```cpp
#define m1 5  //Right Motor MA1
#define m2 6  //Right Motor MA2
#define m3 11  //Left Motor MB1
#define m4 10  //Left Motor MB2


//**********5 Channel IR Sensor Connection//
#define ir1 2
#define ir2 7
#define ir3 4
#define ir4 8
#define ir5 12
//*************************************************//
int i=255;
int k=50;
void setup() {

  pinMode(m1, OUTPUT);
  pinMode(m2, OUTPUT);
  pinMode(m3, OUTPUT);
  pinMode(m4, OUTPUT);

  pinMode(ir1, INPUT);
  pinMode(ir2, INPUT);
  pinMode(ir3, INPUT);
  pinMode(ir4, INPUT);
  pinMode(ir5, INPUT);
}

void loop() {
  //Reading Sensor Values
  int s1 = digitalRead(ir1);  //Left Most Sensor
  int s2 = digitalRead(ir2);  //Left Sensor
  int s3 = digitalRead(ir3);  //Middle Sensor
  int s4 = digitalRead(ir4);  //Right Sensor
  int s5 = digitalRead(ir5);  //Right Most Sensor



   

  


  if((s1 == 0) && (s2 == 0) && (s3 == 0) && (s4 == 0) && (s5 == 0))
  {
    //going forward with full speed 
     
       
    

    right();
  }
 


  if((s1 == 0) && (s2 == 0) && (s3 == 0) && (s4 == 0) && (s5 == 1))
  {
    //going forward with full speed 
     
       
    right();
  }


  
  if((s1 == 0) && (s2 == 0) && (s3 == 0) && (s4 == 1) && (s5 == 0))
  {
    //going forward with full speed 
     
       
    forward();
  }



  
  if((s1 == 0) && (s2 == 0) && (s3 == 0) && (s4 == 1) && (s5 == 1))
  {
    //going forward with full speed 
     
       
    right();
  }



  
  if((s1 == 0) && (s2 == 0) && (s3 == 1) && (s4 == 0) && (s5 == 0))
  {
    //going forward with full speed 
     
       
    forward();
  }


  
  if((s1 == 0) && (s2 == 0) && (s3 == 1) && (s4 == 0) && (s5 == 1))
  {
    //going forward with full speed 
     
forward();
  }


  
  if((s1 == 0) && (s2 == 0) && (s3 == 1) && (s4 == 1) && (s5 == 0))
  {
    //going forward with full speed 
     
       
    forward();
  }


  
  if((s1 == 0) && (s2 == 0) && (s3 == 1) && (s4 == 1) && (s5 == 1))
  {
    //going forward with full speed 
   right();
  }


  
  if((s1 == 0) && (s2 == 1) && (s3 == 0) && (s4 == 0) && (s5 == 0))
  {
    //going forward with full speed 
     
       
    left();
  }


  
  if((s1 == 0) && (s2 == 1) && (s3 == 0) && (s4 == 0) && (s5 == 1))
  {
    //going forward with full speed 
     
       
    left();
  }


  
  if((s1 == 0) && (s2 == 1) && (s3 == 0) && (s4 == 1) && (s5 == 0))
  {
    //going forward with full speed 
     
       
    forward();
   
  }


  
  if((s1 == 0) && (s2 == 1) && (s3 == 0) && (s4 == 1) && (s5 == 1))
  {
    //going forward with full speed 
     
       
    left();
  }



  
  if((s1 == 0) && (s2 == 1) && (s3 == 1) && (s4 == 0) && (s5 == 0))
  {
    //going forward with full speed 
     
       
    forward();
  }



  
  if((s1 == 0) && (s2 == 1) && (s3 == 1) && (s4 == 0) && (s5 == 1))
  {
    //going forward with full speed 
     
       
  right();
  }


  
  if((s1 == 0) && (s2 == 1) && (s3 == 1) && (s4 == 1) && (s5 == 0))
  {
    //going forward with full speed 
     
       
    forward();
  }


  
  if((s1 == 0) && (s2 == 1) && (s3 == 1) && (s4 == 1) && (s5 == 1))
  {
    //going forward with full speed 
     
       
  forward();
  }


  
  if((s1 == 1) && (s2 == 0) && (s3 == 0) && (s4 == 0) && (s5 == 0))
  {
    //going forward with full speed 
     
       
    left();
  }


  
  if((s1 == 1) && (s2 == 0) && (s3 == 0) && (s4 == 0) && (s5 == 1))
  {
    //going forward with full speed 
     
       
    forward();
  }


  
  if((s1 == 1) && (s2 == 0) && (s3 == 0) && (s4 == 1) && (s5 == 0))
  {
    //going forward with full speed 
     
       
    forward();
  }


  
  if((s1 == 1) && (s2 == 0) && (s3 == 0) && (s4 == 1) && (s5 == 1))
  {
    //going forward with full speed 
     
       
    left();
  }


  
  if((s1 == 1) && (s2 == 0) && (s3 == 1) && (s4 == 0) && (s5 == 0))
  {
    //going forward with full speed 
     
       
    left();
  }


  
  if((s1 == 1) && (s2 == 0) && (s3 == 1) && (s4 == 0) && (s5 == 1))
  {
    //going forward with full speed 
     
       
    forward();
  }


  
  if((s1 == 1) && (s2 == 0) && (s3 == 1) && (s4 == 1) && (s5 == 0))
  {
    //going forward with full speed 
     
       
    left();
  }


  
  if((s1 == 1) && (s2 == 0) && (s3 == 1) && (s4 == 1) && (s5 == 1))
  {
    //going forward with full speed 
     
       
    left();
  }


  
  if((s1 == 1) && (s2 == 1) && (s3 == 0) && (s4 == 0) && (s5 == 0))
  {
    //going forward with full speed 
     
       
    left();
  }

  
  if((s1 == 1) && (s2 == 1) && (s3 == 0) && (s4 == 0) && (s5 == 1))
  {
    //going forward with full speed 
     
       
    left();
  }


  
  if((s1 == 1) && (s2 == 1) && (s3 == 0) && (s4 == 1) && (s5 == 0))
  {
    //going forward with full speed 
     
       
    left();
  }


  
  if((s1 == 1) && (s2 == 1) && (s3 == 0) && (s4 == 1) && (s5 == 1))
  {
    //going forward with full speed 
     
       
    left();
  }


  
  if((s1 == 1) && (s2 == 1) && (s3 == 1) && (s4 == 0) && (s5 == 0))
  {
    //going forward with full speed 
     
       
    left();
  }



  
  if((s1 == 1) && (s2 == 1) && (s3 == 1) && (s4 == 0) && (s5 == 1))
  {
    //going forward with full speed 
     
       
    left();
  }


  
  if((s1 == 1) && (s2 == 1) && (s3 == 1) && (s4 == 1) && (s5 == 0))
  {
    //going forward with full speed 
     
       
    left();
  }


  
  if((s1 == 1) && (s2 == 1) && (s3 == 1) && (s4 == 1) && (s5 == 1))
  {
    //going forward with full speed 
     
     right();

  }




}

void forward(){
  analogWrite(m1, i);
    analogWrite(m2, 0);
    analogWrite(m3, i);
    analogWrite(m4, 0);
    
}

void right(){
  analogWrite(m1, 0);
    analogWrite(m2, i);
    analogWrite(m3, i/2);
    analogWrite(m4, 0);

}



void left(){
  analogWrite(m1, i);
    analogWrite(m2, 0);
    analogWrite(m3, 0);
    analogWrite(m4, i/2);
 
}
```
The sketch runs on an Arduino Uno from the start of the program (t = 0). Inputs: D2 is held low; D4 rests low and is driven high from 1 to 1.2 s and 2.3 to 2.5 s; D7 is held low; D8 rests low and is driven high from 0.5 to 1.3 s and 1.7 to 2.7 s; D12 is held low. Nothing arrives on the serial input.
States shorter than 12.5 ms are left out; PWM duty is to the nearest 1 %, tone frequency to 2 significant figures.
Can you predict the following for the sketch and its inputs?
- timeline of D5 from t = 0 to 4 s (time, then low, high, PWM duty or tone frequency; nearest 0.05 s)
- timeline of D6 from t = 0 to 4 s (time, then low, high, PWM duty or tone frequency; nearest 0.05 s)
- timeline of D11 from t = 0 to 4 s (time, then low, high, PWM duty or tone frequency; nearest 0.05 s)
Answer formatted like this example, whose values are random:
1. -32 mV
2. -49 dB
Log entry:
1. 0 s low; 0.5 s high; 1.3 s low; 1.7 s high; 2.7 s low
2. 0 s high; 0.5 s low; 1.3 s high; 1.7 s low; 2.7 s high
3. 0 s PWM 50 %; 0.5 s high; 1.3 s PWM 50 %; 1.7 s high; 2.7 s PWM 50 %
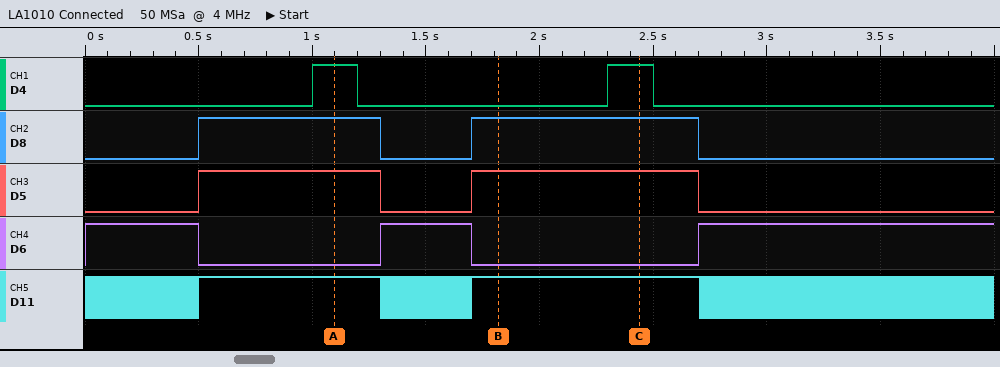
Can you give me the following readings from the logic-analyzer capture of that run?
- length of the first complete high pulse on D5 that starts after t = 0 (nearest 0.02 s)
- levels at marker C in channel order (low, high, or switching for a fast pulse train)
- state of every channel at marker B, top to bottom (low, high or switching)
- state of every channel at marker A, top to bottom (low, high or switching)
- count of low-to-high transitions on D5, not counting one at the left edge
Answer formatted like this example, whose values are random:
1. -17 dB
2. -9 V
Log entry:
1. 0.80 s
2. D4 high, D8 high, D5 high, D6 low, D11 high
3. D4 low, D8 high, D5 high, D6 low, D11 high
4. D4 high, D8 high, D5 high, D6 low, D11 high
5. 2
